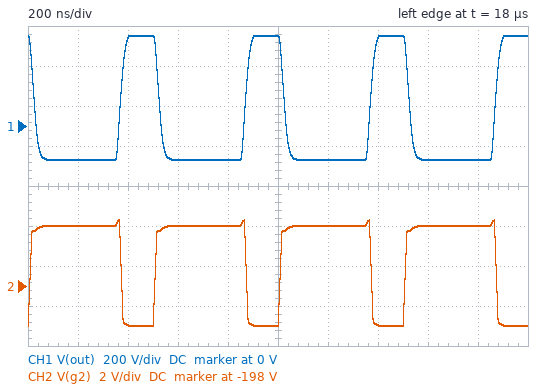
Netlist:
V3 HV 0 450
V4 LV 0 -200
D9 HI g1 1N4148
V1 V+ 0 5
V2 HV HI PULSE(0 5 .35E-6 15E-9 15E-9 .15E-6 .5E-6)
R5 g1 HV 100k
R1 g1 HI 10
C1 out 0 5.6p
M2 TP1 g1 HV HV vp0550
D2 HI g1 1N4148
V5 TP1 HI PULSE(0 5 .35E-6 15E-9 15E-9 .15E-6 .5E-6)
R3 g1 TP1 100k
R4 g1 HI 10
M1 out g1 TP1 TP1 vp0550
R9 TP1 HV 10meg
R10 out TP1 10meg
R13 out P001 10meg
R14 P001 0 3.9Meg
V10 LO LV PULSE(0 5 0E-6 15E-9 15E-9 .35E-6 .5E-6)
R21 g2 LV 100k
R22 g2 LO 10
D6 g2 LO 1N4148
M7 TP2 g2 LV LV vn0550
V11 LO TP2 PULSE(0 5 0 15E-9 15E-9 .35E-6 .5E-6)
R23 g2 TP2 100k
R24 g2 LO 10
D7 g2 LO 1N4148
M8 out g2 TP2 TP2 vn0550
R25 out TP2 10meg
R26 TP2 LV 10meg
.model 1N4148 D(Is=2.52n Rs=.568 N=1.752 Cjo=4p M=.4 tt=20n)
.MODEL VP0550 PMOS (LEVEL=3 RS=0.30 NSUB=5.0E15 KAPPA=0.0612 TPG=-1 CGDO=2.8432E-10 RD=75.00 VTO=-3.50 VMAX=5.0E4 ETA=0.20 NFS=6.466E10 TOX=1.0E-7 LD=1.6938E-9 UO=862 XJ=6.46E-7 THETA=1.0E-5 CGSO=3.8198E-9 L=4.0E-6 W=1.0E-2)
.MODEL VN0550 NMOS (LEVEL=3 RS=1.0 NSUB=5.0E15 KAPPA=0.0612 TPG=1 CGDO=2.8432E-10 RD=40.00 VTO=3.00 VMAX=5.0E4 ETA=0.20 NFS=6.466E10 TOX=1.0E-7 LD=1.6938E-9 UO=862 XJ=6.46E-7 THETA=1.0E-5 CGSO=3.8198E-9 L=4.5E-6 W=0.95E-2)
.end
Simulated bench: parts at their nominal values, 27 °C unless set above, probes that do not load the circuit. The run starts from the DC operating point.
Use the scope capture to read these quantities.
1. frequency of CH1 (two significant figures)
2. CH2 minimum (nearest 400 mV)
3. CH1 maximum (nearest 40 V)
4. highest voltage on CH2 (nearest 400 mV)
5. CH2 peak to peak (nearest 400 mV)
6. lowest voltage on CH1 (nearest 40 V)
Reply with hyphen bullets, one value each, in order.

- 2.0 MHz
- -200.0 V
- 440 V
- -194.8 V
- 5.2 V
- -160 V
